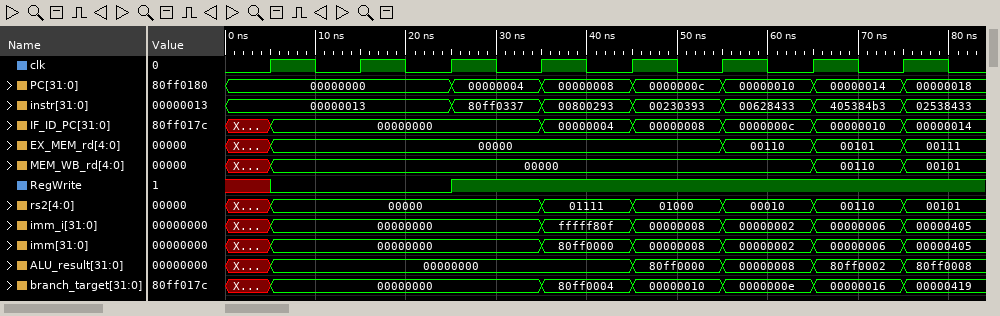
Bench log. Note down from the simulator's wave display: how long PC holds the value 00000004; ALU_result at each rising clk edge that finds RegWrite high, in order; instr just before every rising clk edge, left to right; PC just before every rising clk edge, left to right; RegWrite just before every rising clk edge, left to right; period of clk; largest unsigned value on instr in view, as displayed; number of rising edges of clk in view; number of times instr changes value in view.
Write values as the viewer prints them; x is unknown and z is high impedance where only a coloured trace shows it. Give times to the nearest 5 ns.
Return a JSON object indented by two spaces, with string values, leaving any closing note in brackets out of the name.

{
  "how long PC holds the value 00000004": "10 ns",
  "ALU_result at each rising clk edge that finds RegWrite high, in order": "00000000, 00000000, 80ff0000, 00000008, 80ff0002",
  "instr just before every rising clk edge, left to right": "00000013, 00000013, 00000013, 80ff0337, 00800293, 00230393, 00628433, 405384b3",
  "PC just before every rising clk edge, left to right": "00000000, 00000000, 00000000, 00000004, 00000008, 0000000c, 00000010, 00000014",
  "RegWrite just before every rising clk edge, left to right": "x 0 0 1 1 1 1 1",
  "period of clk": "10 ns",
  "largest unsigned value on instr in view, as displayed": "80ff0337",
  "number of rising edges of clk in view": "8",
  "number of times instr changes value in view": "6"
}
